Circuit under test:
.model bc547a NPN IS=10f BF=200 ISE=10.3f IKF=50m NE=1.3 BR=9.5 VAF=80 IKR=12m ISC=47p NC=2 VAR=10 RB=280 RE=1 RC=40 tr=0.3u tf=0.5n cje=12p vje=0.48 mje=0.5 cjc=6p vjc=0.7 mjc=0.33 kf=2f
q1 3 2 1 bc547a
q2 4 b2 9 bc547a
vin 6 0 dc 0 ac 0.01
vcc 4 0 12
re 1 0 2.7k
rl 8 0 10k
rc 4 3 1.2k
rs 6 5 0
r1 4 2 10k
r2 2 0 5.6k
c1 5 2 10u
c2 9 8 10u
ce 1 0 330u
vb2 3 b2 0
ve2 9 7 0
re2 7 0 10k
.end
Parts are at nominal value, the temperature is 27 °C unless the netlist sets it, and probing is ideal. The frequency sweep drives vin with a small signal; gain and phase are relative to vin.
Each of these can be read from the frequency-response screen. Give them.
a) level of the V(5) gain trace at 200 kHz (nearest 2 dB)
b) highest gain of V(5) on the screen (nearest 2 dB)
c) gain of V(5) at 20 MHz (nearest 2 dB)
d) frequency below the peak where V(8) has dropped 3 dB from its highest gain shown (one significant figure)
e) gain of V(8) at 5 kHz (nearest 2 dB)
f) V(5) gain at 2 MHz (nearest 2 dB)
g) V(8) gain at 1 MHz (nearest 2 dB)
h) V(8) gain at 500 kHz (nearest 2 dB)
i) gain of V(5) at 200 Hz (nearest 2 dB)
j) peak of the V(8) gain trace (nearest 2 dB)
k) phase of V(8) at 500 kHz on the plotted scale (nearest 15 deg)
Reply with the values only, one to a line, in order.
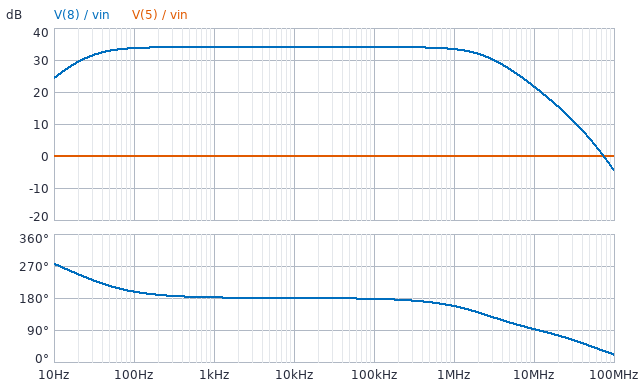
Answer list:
0 dB
0 dB
0 dB
30 Hz
34 dB
0 dB
34 dB
34 dB
0 dB
34 dB
165 deg
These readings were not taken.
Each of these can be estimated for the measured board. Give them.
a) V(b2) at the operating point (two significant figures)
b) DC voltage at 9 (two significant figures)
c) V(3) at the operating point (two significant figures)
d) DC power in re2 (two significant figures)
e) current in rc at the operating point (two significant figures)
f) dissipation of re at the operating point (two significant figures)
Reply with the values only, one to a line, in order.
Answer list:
10 V
9.7 V
10 V
9.5 mW
1.3 mA
4.8 mW
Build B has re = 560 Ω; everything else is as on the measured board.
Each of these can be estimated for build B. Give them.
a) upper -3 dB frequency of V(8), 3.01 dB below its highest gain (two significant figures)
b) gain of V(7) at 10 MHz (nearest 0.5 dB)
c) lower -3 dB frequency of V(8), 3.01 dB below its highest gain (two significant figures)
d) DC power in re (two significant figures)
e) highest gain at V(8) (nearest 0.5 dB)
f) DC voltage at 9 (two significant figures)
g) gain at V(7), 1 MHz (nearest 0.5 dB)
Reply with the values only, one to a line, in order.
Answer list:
690 kHz
19.0 dB
73 Hz
21 mW
42.5 dB
4.1 V
37.5 dB
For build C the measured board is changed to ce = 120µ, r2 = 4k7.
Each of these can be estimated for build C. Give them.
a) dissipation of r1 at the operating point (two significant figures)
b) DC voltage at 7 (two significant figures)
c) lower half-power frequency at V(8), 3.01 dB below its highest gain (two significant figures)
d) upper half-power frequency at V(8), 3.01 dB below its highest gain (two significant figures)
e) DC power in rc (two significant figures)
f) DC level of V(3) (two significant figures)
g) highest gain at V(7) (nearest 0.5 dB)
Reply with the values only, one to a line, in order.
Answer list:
6.7 mW
9.9 V
56 Hz
2.8 MHz
1.6 mW
11 V
33.0 dB
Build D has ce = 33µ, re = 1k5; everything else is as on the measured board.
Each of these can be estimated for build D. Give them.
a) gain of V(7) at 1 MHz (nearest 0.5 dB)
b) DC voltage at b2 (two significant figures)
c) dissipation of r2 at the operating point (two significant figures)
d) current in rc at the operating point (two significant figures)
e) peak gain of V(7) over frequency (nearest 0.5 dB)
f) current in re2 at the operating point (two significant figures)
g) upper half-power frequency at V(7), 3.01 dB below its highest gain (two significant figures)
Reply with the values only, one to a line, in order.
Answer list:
36.5 dB
9.2 V
3.2 mW
2.4 mA
38.0 dB
850 µA
1.7 MHz
